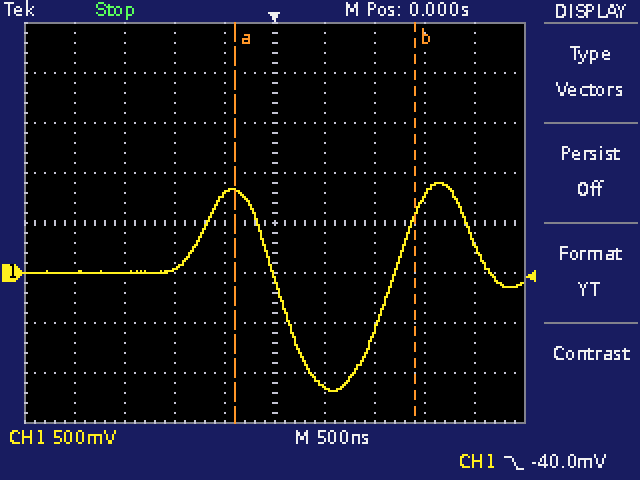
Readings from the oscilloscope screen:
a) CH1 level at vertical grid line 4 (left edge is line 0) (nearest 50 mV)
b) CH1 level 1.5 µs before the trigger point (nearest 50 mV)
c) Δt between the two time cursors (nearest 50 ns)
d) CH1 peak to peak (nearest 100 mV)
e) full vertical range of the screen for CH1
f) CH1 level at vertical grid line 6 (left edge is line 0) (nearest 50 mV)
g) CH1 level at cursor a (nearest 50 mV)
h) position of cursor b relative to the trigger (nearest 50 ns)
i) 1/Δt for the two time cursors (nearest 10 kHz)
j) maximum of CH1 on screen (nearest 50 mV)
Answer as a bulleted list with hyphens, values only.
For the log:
- 800 mV
- 0 mV
- 1.80 µs
- 2.10 V
- 4 V
- -1.15 V
- 800 mV
- +1.40 µs
- 560 kHz
- 900 mV
